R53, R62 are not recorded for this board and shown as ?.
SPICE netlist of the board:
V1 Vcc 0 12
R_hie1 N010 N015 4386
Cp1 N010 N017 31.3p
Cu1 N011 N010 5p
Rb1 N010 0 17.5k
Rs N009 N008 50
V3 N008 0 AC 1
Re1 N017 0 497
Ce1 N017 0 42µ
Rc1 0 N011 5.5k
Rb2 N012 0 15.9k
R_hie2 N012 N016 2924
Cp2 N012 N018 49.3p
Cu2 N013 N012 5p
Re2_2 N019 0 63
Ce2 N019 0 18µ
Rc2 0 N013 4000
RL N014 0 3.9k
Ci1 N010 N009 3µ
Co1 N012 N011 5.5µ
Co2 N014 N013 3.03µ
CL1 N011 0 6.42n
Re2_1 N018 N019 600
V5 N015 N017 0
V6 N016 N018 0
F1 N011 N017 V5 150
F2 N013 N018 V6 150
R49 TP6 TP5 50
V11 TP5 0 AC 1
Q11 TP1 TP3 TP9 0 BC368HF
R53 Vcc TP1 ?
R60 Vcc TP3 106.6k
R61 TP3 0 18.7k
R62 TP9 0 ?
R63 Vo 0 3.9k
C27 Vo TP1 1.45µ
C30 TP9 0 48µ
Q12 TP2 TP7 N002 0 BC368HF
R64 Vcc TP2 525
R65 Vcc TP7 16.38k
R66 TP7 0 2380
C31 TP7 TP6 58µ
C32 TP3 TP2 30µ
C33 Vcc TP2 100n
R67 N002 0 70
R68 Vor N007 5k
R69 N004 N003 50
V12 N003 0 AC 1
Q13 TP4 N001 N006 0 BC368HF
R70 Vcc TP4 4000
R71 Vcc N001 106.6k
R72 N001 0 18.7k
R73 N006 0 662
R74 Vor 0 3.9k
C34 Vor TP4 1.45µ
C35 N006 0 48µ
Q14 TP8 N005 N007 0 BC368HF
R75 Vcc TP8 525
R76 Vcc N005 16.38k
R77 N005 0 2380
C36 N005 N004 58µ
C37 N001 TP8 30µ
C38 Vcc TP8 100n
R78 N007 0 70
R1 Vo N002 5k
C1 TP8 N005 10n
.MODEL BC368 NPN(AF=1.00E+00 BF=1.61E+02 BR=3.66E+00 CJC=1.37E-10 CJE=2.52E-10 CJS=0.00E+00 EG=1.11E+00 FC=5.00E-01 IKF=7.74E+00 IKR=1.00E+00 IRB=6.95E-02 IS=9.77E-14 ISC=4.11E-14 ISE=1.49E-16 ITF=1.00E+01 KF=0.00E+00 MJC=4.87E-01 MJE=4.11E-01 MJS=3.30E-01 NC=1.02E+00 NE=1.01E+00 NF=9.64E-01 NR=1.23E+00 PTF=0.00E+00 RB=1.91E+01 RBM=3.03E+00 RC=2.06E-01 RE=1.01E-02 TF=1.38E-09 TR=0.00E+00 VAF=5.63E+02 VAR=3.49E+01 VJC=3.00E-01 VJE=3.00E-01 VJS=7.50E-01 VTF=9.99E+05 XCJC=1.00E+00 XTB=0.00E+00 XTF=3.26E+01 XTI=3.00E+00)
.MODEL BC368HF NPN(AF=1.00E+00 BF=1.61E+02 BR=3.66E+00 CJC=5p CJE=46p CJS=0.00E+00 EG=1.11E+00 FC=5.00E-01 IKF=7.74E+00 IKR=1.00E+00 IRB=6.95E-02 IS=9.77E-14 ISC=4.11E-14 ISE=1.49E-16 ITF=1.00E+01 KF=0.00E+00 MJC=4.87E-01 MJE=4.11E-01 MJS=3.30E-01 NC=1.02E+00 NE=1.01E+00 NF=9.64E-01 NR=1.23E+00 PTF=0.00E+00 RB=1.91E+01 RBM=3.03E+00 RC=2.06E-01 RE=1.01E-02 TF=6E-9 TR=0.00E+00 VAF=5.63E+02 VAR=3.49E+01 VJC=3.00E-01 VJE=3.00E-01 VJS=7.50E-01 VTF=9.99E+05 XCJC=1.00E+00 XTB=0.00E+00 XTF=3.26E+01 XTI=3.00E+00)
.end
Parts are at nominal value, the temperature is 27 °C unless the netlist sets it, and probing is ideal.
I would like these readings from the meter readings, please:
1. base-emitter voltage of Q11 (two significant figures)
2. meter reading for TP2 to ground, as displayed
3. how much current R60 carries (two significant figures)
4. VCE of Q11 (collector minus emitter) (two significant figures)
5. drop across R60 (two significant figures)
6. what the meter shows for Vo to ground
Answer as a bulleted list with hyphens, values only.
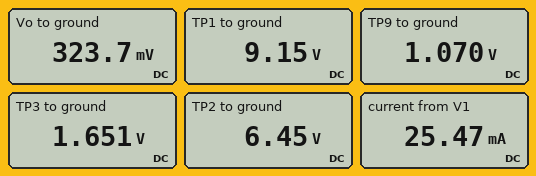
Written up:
- 580 mV
- 6.45 V
- 97 µA
- 8.1 V
- 10 V
- 323.7 mV
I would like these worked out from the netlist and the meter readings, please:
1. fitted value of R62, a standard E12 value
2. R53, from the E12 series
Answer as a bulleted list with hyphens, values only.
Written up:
- 820 Ω
- 2.2 kΩ
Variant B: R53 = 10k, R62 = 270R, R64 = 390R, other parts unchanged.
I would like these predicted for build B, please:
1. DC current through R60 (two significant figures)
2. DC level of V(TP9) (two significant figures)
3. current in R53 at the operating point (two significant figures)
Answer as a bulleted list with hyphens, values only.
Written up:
- 100 µA
- 330 mV
- 1.2 mA
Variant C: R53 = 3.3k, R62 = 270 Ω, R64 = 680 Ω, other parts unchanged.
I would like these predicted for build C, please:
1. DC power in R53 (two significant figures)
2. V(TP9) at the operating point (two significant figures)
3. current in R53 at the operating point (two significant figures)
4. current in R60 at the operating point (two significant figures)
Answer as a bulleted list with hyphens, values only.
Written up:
- 32 mW
- 850 mV
- 3.1 mA
- 99 µA
